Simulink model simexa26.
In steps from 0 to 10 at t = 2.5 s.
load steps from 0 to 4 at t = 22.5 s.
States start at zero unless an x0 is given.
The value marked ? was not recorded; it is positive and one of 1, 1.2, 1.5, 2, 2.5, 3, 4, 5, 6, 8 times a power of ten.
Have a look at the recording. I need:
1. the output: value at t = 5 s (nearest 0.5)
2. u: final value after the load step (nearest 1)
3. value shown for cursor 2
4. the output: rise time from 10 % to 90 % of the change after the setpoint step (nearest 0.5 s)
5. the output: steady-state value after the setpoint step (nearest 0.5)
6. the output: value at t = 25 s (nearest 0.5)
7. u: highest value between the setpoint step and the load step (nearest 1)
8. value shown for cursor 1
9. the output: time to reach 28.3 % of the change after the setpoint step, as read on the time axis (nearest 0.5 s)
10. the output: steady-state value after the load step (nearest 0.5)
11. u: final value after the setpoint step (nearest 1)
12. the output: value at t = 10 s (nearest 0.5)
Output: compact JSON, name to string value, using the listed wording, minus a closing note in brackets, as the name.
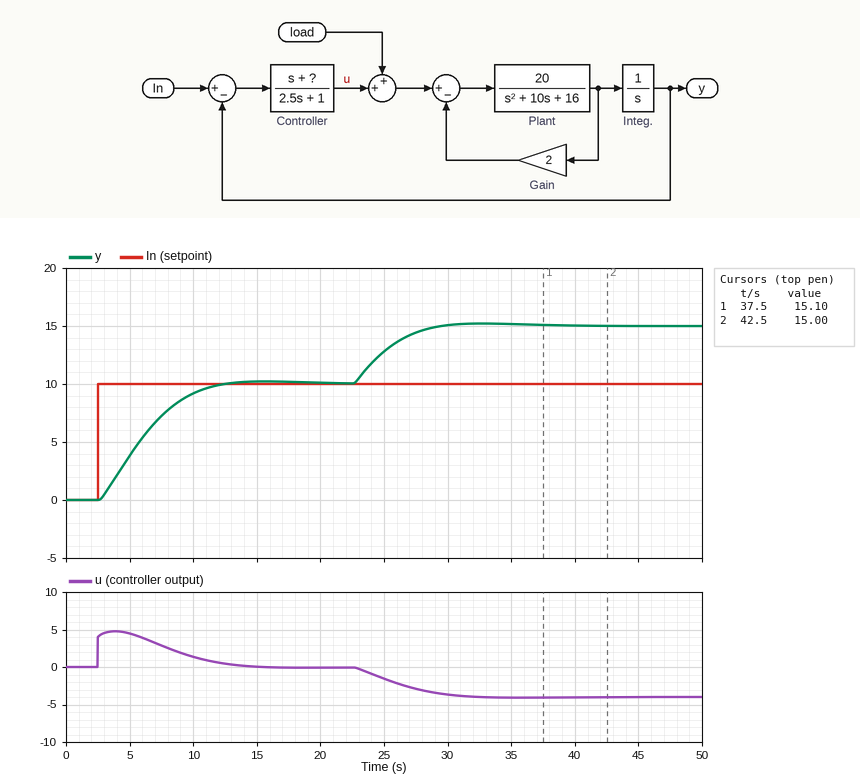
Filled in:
{"the output: value at t = 5 s": "4.0", "u: final value after the load step": "-4", "value shown for cursor 2": "15.00", "the output: rise time from 10 % to 90 % of the change after the setpoint step": "6.5 s", "the output: steady-state value after the setpoint step": "10.0", "the output: value at t = 25 s": "13.0", "u: highest value between the setpoint step and the load step": "5", "value shown for cursor 1": "15.10", "the output: time to reach 28.3 % of the change after the setpoint step, as read on the time axis": "4.5 s", "the output: steady-state value after the load step": "15.0", "u: final value after the setpoint step": "0", "the output: value at t = 10 s": "9.0"}
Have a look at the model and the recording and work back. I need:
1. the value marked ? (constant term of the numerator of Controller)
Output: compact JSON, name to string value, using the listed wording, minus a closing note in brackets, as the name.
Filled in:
{"the value marked ?": "0.8"}
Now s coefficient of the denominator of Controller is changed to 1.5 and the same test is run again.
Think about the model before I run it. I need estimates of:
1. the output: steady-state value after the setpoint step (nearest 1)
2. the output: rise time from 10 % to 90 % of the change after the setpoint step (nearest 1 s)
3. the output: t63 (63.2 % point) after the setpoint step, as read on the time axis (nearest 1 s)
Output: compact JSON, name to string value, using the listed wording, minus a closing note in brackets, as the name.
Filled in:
{"the output: steady-state value after the setpoint step": "10", "the output: rise time from 10 % to 90 % of the change after the setpoint step": "7 s", "the output: t63 (63.2 % point) after the setpoint step, as read on the time axis": "6 s"}
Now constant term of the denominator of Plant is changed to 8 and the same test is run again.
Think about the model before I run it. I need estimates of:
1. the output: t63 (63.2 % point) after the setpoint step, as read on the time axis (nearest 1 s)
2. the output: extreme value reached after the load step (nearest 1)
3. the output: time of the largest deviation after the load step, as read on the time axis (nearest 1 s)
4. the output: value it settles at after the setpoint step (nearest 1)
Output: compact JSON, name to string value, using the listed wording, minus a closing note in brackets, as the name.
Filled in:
{"the output: t63 (63.2 % point) after the setpoint step, as read on the time axis": "6 s", "the output: extreme value reached after the load step": "15", "the output: time of the largest deviation after the load step, as read on the time axis": "31 s", "the output: value it settles at after the setpoint step": "10"}
